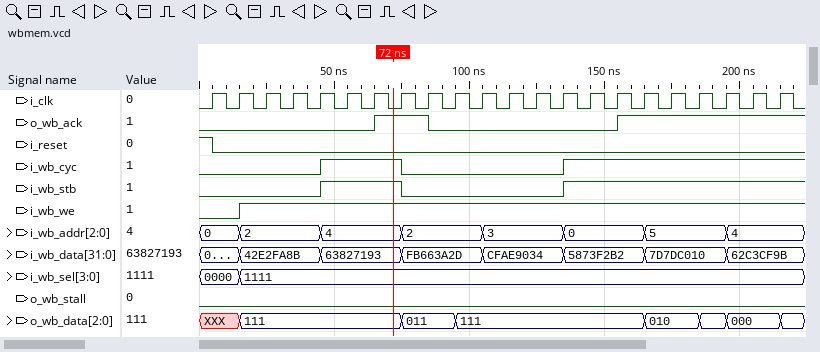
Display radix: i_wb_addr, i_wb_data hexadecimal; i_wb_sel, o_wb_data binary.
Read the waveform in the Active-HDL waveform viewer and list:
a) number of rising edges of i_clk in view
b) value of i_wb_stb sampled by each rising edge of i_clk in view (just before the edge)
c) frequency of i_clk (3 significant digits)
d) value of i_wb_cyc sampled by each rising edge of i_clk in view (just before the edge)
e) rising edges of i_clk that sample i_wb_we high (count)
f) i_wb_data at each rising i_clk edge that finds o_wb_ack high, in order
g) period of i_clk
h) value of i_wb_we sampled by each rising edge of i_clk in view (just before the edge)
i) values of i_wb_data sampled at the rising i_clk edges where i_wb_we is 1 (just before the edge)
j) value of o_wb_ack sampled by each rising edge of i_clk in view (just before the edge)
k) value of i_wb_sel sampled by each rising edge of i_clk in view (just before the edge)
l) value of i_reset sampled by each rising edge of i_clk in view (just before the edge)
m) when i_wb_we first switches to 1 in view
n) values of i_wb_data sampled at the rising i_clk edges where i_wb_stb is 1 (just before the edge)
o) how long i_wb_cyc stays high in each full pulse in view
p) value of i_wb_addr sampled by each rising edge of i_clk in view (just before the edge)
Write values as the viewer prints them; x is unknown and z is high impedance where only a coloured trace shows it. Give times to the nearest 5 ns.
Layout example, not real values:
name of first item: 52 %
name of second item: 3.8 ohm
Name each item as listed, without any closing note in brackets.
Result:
number of rising edges of i_clk in view: 22
value of i_wb_stb sampled by each rising edge of i_clk in view: 0 0 0 0 0 1 1 1 0 0 0 0 0 0 1 1 1 1 1 1 1 1
frequency of i_clk: 100 MHz
value of i_wb_cyc sampled by each rising edge of i_clk in view: 0 0 0 0 0 1 1 1 0 0 0 0 0 0 1 1 1 1 1 1 1 1
rising edges of i_clk that sample i_wb_we high: 20
i_wb_data at each rising i_clk edge that finds o_wb_ack high, in order: 63827193, FB663A2D, 5873F2B2, 7D7DC010, 7D7DC010, 7D7DC010, 62C3CF9B, 62C3CF9B
period of i_clk: 10 ns
value of i_wb_we sampled by each rising edge of i_clk in view: 0 0 1 1 1 1 1 1 1 1 1 1 1 1 1 1 1 1 1 1 1 1
values of i_wb_data sampled at the rising i_clk edges where i_wb_we is 1: 42E2FA8B, 42E2FA8B, 42E2FA8B, 63827193, 63827193, 63827193, FB663A2D, FB663A2D, FB663A2D, CFAE9034, CFAE9034, CFAE9034, 5873F2B2, 5873F2B2, 5873F2B2, 7D7DC010, 7D7DC010, 7D7DC010, 62C3CF9B, 62C3CF9B
value of o_wb_ack sampled by each rising edge of i_clk in view: 0 0 0 0 0 0 0 1 1 0 0 0 0 0 0 0 1 1 1 1 1 1
value of i_wb_sel sampled by each rising edge of i_clk in view: 0000, 0000, 1111, 1111, 1111, 1111, 1111, 1111, 1111, 1111, 1111, 1111, 1111, 1111, 1111, 1111, 1111, 1111, 1111, 1111, 1111, 1111
value of i_reset sampled by each rising edge of i_clk in view: 1 0 0 0 0 0 0 0 0 0 0 0 0 0 0 0 0 0 0 0 0 0
when i_wb_we first switches to 1 in view: 15 ns
values of i_wb_data sampled at the rising i_clk edges where i_wb_stb is 1: 63827193, 63827193, 63827193, 5873F2B2, 5873F2B2, 5873F2B2, 7D7DC010, 7D7DC010, 7D7DC010, 62C3CF9B, 62C3CF9B
how long i_wb_cyc stays high in each full pulse in view: 30 ns
value of i_wb_addr sampled by each rising edge of i_clk in view: 0, 0, 2, 2, 2, 4, 4, 4, 2, 2, 2, 3, 3, 3, 0, 0, 0, 5, 5, 5, 4, 4
